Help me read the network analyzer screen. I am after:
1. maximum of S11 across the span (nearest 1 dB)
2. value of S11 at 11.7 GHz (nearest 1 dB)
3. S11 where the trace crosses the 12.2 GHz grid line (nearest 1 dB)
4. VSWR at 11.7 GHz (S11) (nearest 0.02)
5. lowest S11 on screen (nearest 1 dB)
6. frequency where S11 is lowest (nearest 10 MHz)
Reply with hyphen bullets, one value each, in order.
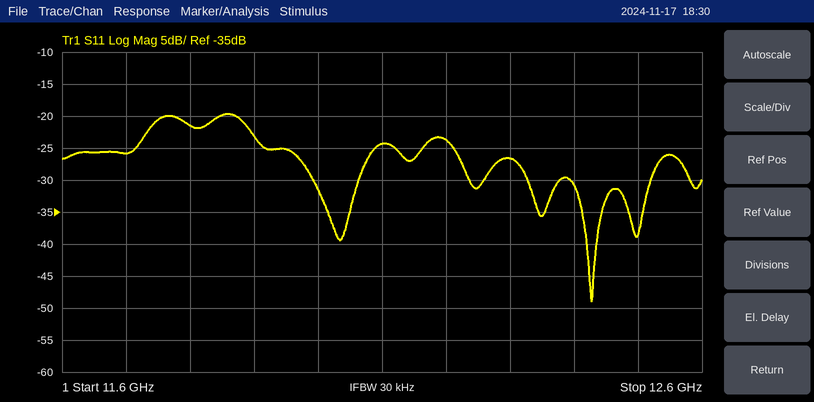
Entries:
- -20 dB
- -26 dB
- -24 dB
- 1.10
- -49 dB
- 12.43 GHz
